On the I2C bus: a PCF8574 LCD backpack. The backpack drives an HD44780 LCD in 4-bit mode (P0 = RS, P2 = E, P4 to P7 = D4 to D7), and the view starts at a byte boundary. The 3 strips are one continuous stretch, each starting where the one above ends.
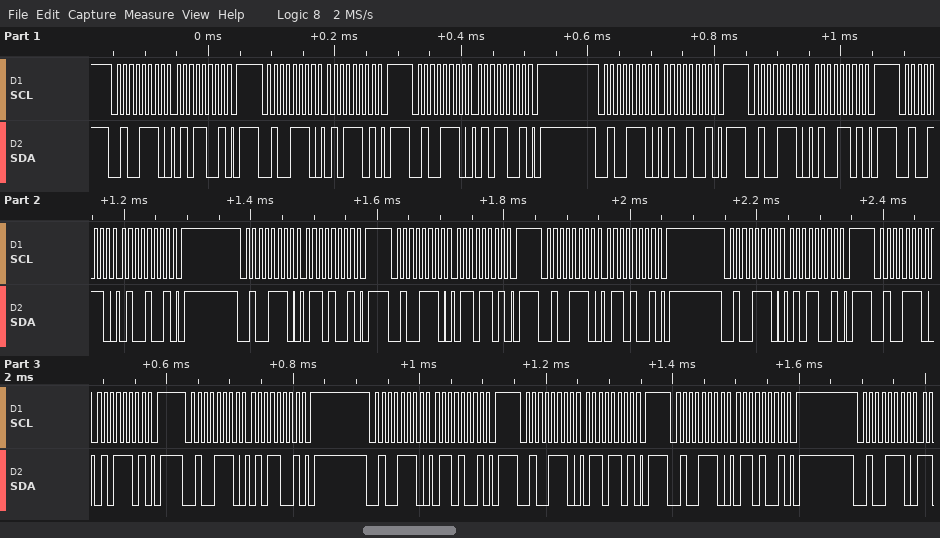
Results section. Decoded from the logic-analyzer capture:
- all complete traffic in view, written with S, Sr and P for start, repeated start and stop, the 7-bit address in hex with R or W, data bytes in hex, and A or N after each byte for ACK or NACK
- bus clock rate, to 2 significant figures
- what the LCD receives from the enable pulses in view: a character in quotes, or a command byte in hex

S 27W A 59 A P S 27W A 5D A P S 27W A 59 A P S 27W A 49 A P S 27W A 4D A P S 27W A 49 A P S 27W A 69 A P S 27W A 6D A P S 27W A 69 A P S 27W A 59 A P S 27W A 5D A P S 27W A 59 A P S 27W A 69 A P S 27W A 6D A P S 27W A 69 A P S 27W A
100 kHz
'T' 'e'
